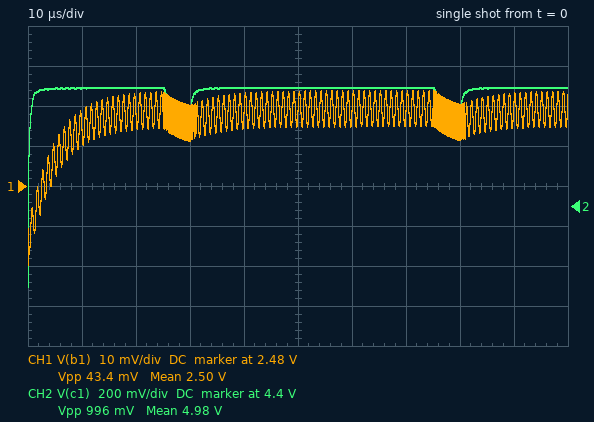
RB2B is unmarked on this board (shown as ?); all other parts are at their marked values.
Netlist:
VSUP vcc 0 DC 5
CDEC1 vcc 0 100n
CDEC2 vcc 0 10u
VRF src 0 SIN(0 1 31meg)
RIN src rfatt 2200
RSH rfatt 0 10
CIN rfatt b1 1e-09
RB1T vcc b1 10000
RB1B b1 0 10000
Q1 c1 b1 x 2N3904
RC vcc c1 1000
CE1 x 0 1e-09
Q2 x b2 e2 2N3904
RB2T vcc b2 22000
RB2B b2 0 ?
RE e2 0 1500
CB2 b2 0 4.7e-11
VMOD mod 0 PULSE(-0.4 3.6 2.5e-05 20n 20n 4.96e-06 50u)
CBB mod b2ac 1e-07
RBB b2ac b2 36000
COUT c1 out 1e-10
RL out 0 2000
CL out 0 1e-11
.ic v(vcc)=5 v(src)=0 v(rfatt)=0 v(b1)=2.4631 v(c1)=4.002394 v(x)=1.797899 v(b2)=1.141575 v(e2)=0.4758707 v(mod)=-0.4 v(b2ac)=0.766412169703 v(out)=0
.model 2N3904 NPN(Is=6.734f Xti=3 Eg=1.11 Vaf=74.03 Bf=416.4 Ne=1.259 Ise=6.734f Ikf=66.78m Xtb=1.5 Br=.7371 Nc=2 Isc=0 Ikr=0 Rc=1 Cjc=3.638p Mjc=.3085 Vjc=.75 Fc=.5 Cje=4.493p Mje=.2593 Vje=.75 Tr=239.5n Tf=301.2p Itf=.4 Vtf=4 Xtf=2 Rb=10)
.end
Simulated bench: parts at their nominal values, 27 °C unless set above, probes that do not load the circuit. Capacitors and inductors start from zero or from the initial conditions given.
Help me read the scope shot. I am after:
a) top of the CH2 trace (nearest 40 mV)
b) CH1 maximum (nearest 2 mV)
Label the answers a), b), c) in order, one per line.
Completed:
a) 5.00 V
b) 2.504 V
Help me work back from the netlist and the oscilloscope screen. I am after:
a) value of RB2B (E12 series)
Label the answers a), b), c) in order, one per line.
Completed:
a) 2.7 kΩ
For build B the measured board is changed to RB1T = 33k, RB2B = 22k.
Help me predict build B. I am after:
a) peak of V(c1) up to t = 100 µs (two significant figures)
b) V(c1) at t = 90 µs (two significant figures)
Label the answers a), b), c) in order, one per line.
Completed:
a) 4.9 V
b) 4.8 V
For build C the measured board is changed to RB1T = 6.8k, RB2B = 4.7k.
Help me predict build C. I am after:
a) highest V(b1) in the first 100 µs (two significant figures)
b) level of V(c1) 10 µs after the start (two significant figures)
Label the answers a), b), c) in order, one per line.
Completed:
a) 3.0 V
b) 4.8 V
